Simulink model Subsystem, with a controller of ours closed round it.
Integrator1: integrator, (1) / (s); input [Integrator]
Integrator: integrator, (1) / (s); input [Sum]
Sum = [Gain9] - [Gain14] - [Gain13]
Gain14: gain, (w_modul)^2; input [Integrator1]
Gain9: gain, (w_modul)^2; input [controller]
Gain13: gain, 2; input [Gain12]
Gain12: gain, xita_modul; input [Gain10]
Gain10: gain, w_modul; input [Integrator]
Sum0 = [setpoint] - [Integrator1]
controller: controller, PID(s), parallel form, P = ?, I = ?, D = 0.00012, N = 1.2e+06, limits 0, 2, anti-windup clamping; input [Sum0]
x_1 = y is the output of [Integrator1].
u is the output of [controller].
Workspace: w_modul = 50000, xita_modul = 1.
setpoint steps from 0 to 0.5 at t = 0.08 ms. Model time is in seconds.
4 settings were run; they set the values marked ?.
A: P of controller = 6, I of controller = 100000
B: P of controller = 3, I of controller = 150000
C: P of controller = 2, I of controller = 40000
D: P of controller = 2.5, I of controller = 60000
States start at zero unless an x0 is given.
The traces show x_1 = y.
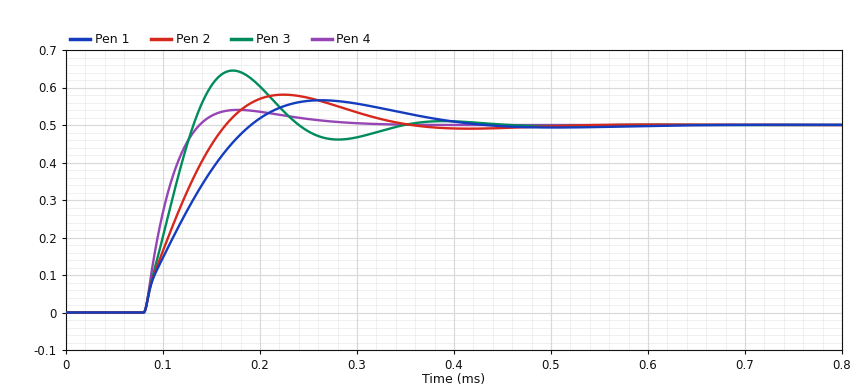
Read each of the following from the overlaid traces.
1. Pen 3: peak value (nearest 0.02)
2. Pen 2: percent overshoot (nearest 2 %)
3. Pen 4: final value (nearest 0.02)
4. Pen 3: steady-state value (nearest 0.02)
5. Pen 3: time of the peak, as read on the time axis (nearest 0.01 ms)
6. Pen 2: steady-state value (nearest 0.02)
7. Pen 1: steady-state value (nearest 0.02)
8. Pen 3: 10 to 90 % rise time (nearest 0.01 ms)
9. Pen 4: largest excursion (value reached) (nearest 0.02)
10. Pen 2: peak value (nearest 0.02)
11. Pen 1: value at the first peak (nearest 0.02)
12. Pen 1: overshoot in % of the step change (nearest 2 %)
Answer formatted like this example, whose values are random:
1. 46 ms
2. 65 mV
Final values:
1. 0.64
2. 16 %
3. 0.50
4. 0.50
5. 0.17 ms
6. 0.50
7. 0.50
8. 0.04 ms
9. 0.54
10. 0.58
11. 0.56
12. 14 %
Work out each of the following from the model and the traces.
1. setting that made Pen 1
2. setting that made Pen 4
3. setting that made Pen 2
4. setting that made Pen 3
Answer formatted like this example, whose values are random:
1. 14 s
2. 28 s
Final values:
1. C
2. A
3. D
4. B
